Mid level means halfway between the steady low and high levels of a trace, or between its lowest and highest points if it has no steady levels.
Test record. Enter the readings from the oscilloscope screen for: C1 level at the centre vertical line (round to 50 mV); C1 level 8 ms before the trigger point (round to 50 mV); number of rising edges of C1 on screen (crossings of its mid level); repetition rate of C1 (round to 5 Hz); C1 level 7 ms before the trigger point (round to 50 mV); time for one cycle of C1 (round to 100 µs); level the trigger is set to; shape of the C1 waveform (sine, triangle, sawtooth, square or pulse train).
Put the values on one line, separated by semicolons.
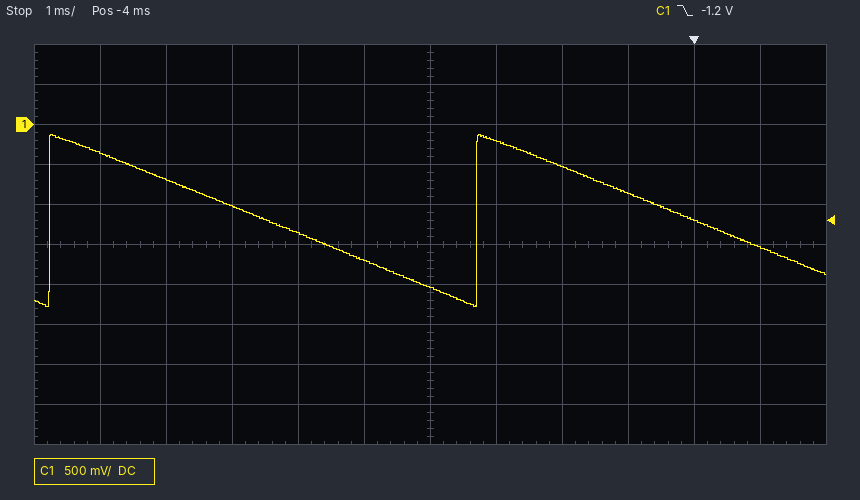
-2.05 V; -700 mV; 2; 155 Hz; -1.00 V; 6.5 ms; -1.2 V; sawtooth
